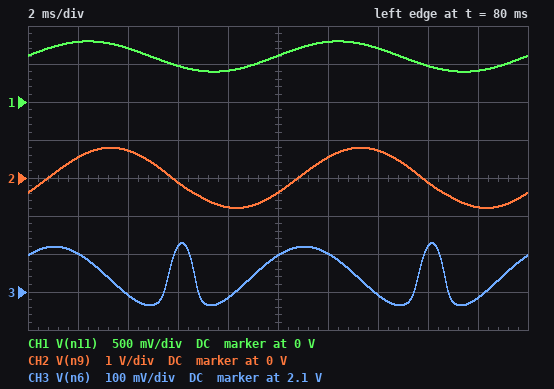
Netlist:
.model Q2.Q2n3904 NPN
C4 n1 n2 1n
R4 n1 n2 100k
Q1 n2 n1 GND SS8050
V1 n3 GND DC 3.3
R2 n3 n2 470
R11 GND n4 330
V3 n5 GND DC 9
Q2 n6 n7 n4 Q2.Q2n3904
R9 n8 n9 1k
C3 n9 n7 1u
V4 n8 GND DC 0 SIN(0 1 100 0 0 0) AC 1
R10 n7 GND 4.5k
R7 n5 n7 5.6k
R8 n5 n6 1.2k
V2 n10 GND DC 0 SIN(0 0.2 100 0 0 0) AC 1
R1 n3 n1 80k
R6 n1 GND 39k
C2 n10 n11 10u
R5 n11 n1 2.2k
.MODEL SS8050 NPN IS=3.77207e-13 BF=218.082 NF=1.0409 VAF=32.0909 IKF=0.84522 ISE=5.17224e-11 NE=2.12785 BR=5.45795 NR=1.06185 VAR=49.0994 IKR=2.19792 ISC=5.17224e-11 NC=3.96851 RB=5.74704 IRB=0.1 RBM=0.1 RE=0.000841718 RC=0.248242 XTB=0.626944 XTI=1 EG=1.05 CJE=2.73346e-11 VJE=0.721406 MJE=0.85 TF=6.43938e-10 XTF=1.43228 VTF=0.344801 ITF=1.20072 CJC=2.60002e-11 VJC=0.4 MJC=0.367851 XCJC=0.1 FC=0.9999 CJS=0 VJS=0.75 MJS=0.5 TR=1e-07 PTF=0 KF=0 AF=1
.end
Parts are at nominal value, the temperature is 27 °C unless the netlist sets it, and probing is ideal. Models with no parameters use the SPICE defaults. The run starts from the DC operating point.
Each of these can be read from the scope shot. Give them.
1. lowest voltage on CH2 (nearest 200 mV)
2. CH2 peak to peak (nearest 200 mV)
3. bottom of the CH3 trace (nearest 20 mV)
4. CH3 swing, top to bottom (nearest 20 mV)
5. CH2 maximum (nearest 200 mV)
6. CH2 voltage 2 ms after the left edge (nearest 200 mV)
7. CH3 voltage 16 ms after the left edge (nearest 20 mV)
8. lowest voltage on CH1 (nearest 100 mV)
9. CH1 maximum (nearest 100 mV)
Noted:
-800 mV
1.6 V
2.06 V
160 mV
800 mV
600 mV
2.22 V
400 mV
800 mV
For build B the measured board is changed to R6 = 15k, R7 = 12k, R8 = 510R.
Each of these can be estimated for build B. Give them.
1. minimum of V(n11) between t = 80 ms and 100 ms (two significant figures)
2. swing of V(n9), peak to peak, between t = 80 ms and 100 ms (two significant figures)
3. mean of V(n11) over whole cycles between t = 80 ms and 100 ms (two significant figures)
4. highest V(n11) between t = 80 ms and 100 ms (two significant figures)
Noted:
360 mV
1.6 V
560 mV
760 mV
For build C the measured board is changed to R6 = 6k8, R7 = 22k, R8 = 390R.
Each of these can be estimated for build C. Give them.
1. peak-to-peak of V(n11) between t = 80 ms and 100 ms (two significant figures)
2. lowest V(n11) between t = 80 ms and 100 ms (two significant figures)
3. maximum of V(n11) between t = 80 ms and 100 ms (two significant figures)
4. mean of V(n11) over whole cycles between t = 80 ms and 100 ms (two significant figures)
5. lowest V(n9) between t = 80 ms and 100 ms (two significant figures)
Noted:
400 mV
230 mV
630 mV
430 mV
-800 mV
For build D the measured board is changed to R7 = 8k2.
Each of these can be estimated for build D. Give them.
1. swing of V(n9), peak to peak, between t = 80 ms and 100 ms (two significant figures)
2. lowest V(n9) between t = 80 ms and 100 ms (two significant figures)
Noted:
1.5 V
-720 mV
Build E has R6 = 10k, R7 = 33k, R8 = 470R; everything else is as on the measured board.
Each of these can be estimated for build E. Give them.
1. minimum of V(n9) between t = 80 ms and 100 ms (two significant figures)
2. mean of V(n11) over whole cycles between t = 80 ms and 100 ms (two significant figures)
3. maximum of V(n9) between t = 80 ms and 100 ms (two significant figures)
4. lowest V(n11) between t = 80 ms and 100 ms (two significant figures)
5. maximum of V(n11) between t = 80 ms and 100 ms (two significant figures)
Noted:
-810 mV
520 mV
810 mV
320 mV
720 mV
